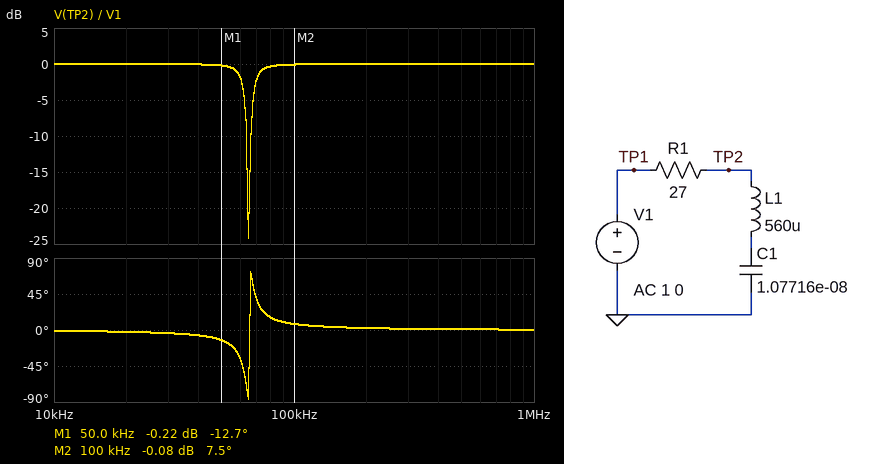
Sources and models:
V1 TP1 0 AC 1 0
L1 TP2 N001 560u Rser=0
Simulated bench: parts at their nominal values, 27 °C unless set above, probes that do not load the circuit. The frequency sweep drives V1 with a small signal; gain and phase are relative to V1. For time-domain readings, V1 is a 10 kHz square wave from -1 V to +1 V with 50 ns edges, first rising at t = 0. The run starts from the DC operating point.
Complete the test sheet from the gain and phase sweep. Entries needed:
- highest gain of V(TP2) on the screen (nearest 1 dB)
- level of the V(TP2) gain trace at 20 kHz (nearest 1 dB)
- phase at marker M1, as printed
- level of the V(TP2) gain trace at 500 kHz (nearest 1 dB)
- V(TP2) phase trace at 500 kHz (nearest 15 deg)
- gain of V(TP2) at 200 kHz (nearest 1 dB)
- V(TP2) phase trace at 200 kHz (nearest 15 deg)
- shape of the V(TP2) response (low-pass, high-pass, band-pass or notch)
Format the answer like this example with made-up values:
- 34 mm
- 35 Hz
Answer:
- 0 dB
- 0 dB
- -12.7 deg
- 0 dB
- 0 deg
- 0 dB
- 0 deg
- notch
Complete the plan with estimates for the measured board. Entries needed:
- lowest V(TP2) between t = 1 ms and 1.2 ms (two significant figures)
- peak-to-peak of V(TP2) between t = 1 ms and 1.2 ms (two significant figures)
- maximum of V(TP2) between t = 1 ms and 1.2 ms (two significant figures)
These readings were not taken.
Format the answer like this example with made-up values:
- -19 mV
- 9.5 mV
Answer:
- -1.2 V
- 2.3 V
- 1.2 V
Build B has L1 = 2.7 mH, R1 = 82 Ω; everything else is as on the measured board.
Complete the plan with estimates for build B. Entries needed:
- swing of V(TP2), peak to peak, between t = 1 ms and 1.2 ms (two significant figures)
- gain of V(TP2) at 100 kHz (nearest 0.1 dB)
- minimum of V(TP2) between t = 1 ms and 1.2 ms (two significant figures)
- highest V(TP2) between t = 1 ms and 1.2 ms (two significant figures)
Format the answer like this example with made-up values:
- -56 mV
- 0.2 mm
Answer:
- 2.8 V
- 0 dB
- -1.4 V
- 1.4 V
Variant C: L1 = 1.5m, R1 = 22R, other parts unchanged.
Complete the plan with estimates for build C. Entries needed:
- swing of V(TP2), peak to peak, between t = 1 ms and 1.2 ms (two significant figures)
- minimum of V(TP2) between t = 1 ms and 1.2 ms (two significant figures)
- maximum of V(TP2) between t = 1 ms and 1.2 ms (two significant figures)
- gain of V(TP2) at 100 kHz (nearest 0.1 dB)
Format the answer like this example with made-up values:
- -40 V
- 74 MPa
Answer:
- 2.1 V
- -1.1 V
- 1.1 V
- 0 dB
